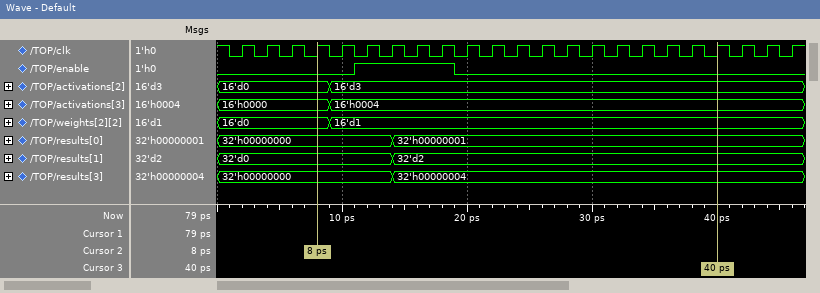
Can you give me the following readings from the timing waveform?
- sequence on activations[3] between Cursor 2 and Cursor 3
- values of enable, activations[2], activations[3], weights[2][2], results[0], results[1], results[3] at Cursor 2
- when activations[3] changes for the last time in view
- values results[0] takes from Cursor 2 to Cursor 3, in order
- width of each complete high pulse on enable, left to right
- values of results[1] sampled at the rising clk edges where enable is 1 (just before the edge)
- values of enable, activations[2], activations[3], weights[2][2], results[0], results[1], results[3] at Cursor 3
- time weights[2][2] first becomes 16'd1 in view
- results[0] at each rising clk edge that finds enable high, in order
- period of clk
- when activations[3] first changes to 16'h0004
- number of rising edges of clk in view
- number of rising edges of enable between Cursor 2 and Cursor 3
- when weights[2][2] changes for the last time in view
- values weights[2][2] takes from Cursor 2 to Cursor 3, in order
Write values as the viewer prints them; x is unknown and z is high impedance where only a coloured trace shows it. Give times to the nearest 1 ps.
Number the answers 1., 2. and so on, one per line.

1. 16'h0000, 16'h0004
2. enable=0, activations[2]=16'd0, activations[3]=16'h0000, weights[2][2]=16'd0, results[0]=32'h00000000, results[1]=32'd0, results[3]=32'h00000000
3. 9 ps
4. 32'h00000000, 32'h00000001
5. 8 ps
6. 32'd0, 32'd0, 32'd2, 32'd2
7. enable=0, activations[2]=16'd3, activations[3]=16'h0004, weights[2][2]=16'd1, results[0]=32'h00000001, results[1]=32'd2, results[3]=32'h00000004
8. 9 ps
9. 32'h00000000, 32'h00000000, 32'h00000001, 32'h00000001
10. 2 ps
11. 9 ps
12. 23
13. 1
14. 9 ps
15. 16'd0, 16'd1
